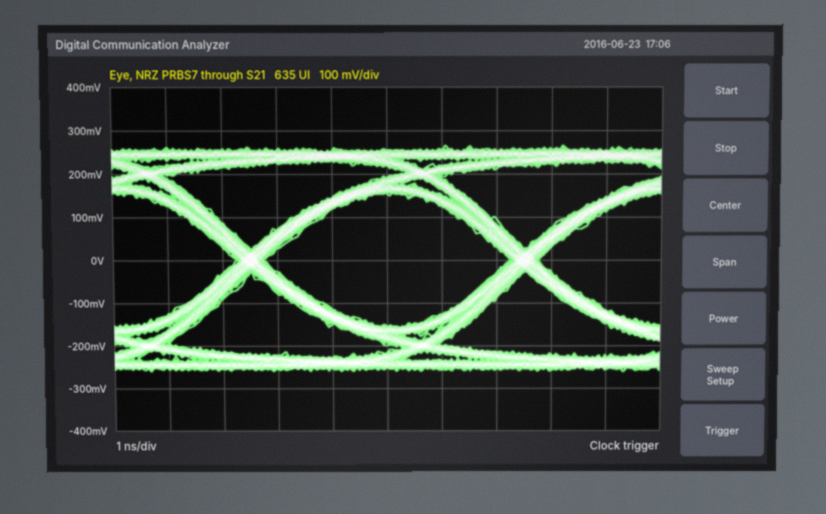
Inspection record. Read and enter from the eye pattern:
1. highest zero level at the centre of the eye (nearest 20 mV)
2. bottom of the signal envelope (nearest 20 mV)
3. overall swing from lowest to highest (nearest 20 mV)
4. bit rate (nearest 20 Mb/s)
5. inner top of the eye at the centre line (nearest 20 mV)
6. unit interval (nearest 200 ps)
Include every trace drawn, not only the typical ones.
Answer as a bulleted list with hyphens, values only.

- -160 mV
- -260 mV
- 520 mV
- 200 Mb/s
- 160 mV
- 5.0 ns
